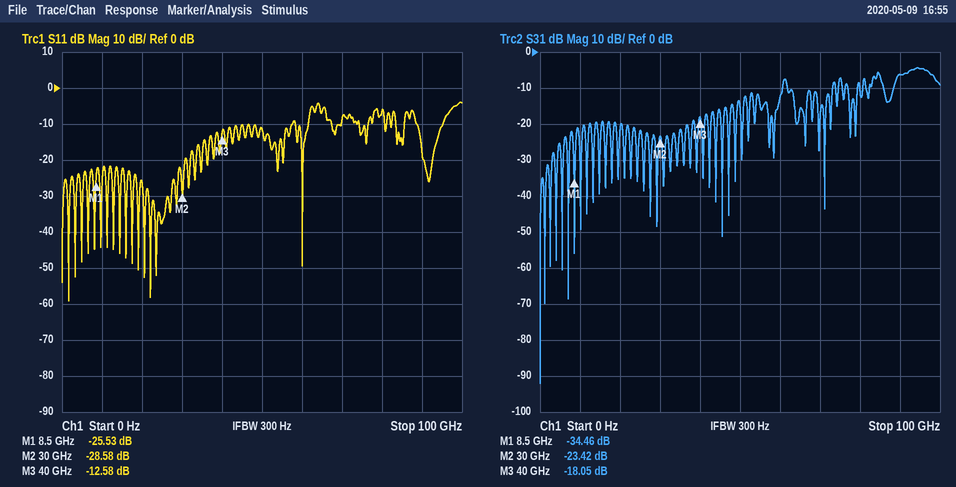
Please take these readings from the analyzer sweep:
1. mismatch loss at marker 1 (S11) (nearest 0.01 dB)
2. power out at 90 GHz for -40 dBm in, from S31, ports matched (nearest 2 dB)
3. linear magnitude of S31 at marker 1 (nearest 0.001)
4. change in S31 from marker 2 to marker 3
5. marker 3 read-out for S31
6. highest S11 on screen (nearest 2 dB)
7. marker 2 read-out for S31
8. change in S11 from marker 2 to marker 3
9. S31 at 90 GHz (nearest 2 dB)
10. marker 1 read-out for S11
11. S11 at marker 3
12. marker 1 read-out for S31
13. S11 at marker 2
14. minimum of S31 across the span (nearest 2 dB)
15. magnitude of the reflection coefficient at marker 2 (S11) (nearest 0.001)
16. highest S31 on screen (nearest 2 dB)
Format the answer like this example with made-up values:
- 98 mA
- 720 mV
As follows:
- 0.01 dB
- -46 dBm
- 0.019
- 5.37 dB
- -18.05 dB
- -4 dB
- -23.42 dB
- 16.00 dB
- -6 dB
- -25.53 dB
- -12.58 dB
- -34.46 dB
- -28.58 dB
- -92 dB
- 0.037
- -4 dB
